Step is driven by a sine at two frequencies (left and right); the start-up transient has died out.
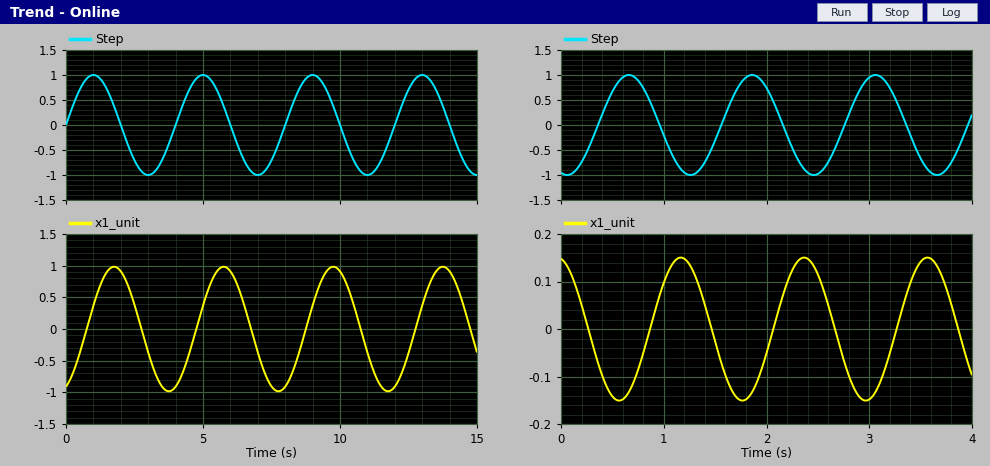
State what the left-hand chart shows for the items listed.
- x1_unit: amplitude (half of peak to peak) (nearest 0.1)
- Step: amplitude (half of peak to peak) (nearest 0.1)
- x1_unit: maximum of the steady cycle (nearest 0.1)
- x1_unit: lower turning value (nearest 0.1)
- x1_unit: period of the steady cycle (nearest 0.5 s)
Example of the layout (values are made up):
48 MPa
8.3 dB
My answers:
1.0
1.0
1.0
-1.0
4.0 s
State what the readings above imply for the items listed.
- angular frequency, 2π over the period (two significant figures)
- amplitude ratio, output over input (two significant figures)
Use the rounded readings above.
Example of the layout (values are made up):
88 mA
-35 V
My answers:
1.6 rad/s
1.0
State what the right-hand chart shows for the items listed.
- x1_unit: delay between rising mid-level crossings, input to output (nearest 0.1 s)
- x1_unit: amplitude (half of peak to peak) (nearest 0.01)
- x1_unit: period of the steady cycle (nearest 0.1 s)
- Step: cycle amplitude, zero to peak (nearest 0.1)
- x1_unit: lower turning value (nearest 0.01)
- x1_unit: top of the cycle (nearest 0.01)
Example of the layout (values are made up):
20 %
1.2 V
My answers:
0.5 s
0.15
1.2 s
1.0
-0.15
0.15
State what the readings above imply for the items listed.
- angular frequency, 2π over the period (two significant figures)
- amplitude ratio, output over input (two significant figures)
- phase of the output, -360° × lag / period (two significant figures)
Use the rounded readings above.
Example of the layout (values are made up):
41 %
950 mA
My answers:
5.2 rad/s
0.15
-150°
